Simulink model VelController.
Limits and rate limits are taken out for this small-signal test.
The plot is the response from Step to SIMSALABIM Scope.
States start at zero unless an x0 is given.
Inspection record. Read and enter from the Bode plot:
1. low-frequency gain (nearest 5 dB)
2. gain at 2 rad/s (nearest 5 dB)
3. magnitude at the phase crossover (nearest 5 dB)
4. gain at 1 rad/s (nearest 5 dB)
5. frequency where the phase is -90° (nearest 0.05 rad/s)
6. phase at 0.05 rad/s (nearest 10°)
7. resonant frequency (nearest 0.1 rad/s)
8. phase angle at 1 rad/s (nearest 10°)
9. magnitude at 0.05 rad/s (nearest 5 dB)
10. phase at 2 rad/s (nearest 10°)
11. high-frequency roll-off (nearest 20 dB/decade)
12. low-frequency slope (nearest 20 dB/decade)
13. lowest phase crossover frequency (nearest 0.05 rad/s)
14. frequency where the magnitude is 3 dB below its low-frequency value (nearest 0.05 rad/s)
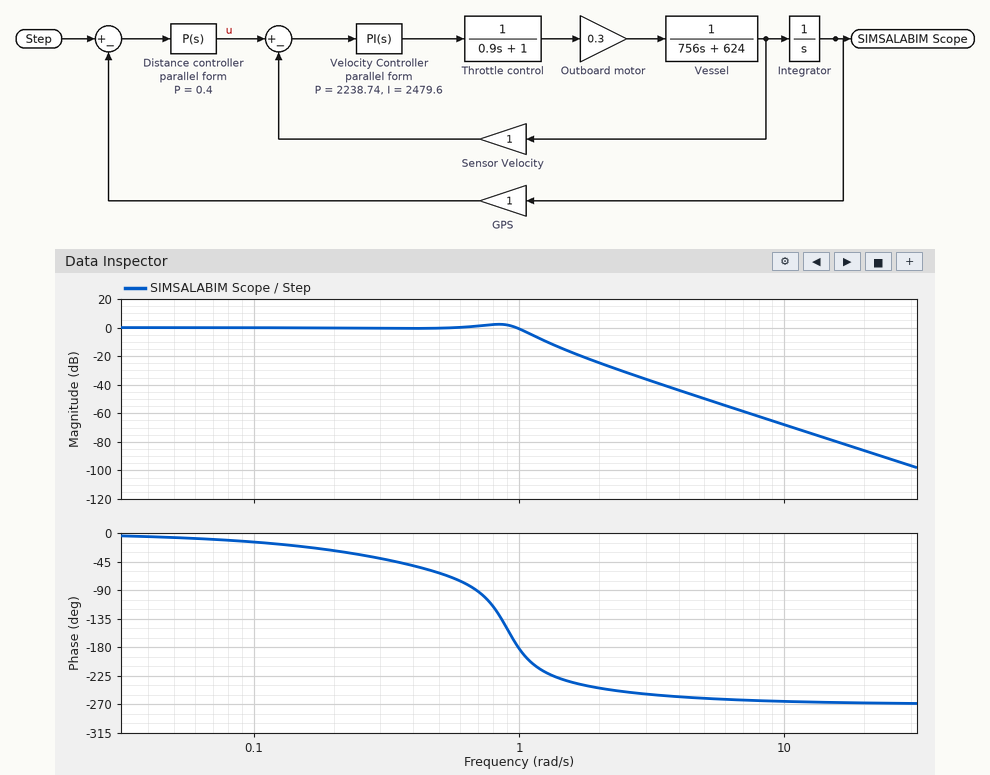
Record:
0 dB
-25 dB
0 dB
0 dB
0.70 rad/s
-10°
0.8 rad/s
-180°
0 dB
-240°
-60 dB/decade
0 dB/decade
1.00 rad/s
1.05 rad/s
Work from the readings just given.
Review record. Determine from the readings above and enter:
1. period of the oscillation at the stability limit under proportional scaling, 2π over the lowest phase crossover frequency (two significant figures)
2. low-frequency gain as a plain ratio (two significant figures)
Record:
6.3 s
1.0
